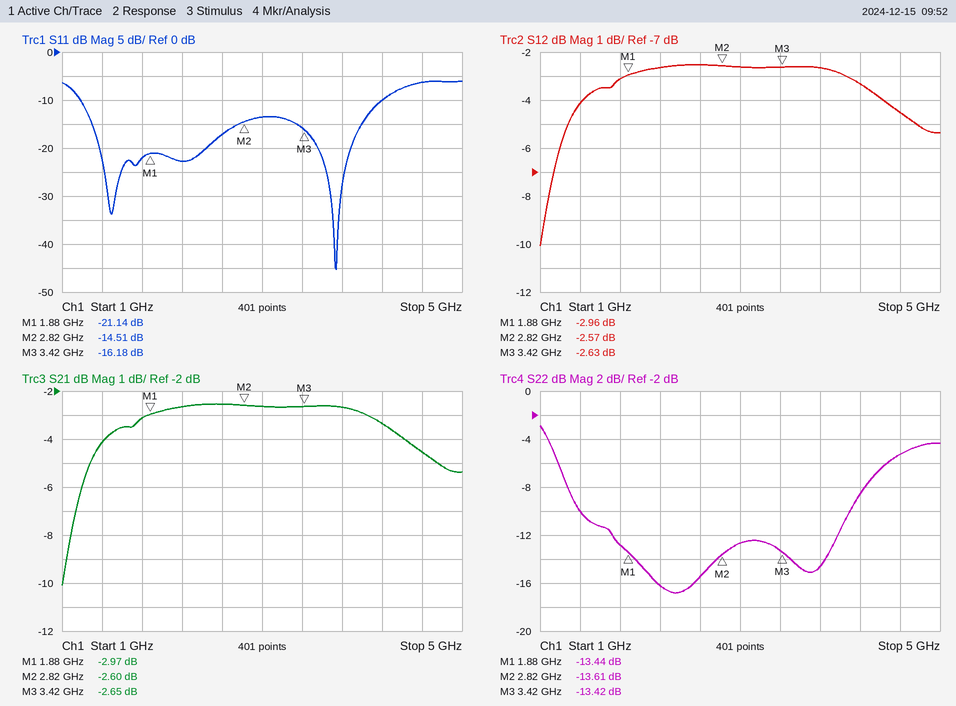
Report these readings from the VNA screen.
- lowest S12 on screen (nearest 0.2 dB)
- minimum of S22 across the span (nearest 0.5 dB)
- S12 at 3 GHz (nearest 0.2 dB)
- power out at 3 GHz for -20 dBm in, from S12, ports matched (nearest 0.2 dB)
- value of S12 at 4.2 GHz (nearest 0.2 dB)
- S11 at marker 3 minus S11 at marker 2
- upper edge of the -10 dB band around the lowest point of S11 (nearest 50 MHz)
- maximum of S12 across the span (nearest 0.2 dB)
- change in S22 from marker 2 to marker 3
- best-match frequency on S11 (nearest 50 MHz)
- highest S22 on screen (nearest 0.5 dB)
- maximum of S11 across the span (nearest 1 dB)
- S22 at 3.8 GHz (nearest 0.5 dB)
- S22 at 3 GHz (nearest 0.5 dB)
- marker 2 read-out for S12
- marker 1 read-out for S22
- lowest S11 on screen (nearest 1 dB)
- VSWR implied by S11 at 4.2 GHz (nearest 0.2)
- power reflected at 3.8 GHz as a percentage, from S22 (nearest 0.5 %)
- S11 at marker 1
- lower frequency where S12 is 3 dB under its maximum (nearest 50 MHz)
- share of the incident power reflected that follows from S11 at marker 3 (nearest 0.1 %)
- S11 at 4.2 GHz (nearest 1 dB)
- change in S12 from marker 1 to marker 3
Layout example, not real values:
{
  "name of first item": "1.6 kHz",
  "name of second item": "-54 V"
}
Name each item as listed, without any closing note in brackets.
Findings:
{
  "lowest S12 on screen": "-10.0 dB",
  "minimum of S22 across the span": "-17.0 dB",
  "S12 at 3 GHz": "-2.6 dB",
  "power out at 3 GHz for -20 dBm in, from S12, ports matched": "-22.6 dBm",
  "value of S12 at 4.2 GHz": "-3.4 dB",
  "S11 at marker 3 minus S11 at marker 2": "-1.67 dB",
  "upper edge of the -10 dB band around the lowest point of S11": "4.20 GHz",
  "maximum of S12 across the span": "-2.6 dB",
  "change in S22 from marker 2 to marker 3": "0.19 dB",
  "best-match frequency on S11": "3.75 GHz",
  "highest S22 on screen": "-3.0 dB",
  "maximum of S11 across the span": "-6 dB",
  "S22 at 3.8 GHz": "-14.5 dB",
  "S22 at 3 GHz": "-12.5 dB",
  "marker 2 read-out for S12": "-2.57 dB",
  "marker 1 read-out for S22": "-13.44 dB",
  "lowest S11 on screen": "-45 dB",
  "VSWR implied by S11 at 4.2 GHz": "2.0",
  "power reflected at 3.8 GHz as a percentage, from S22": "3.5 %",
  "S11 at marker 1": "-21.14 dB",
  "lower frequency where S12 is 3 dB under its maximum": "1.25 GHz",
  "share of the incident power reflected that follows from S11 at marker 3": "2.4 %",
  "S11 at 4.2 GHz": "-10 dB",
  "change in S12 from marker 1 to marker 3": "0.33 dB"
}
